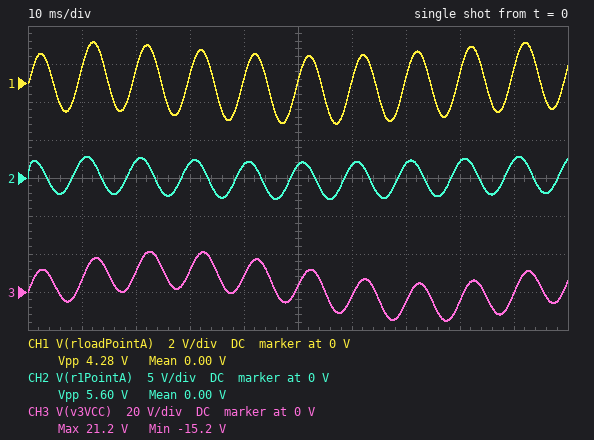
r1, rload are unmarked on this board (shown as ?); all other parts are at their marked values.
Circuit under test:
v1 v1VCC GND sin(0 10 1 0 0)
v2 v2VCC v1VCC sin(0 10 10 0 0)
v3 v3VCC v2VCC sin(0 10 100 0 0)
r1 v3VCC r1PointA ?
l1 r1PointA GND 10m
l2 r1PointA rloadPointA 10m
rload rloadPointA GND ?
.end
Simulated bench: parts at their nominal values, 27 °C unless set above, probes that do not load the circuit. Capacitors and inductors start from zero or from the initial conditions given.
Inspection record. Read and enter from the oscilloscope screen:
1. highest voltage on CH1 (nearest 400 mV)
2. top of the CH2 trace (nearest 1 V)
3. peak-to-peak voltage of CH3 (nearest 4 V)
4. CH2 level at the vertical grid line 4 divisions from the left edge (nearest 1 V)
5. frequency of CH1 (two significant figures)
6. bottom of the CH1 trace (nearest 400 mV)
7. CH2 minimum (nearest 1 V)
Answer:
2.0 V
3 V
36 V
2 V
100 Hz
-2.0 V
-3 V
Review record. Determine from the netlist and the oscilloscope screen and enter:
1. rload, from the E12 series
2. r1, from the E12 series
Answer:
6.8 Ω
15 Ω
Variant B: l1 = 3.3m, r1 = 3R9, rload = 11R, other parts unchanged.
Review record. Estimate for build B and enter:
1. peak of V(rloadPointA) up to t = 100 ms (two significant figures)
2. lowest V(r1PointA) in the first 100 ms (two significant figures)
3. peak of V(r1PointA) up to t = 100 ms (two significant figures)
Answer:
4.1 V
-4.6 V
4.7 V
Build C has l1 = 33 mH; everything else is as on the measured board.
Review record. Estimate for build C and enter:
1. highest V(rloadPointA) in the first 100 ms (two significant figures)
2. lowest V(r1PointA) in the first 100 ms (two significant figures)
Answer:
3.5 V
-4.6 V
